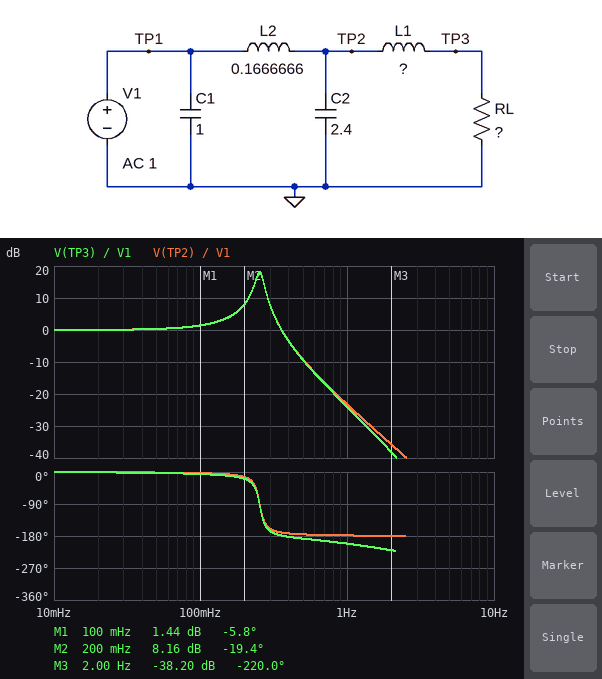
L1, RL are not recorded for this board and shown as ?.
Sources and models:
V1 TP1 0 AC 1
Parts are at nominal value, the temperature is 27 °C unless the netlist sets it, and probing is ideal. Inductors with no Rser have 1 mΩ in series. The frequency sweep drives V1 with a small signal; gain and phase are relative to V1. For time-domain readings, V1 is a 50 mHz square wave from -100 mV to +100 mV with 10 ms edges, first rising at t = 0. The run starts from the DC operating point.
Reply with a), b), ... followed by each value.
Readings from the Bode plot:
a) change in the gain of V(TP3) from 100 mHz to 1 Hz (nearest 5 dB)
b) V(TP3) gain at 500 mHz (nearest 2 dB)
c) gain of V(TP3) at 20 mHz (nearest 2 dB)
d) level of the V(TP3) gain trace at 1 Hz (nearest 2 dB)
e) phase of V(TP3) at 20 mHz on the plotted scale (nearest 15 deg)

a) -25 dB
b) -10 dB
c) 0 dB
d) -24 dB
e) 0 deg
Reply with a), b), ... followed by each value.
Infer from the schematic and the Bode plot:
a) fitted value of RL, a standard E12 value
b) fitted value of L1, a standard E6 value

a) 2.2 Ω
b) 150 mH
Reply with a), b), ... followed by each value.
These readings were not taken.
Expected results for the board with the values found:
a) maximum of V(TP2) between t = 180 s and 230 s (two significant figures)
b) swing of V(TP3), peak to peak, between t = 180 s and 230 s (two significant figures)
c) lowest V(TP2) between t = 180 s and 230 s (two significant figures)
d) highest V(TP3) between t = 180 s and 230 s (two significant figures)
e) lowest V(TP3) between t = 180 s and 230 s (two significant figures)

a) 360 mV
b) 720 mV
c) -360 mV
d) 360 mV
e) -360 mV
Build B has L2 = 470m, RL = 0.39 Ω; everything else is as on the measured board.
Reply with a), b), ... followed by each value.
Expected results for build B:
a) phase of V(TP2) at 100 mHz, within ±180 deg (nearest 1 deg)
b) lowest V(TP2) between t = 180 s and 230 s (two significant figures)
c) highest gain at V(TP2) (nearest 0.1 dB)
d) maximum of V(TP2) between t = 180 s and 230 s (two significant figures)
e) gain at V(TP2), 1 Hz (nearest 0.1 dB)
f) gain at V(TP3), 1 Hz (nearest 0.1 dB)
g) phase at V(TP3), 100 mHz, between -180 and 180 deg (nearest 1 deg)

a) -44 deg
b) -110 mV
c) 0 dB
d) 110 mV
e) -32.2 dB
f) -40.6 dB
g) -58 deg
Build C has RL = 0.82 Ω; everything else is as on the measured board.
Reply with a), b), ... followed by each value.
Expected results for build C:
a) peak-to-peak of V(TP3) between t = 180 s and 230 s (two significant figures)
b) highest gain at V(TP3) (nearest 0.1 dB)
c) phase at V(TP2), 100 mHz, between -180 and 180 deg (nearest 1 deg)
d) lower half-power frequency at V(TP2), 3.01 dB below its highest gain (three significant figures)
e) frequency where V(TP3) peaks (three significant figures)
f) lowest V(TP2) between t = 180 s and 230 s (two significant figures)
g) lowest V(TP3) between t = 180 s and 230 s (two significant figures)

a) 450 mV
b) 9.8 dB
c) -8 deg
d) 212 mHz
e) 257 mHz
f) -230 mV
g) -220 mV
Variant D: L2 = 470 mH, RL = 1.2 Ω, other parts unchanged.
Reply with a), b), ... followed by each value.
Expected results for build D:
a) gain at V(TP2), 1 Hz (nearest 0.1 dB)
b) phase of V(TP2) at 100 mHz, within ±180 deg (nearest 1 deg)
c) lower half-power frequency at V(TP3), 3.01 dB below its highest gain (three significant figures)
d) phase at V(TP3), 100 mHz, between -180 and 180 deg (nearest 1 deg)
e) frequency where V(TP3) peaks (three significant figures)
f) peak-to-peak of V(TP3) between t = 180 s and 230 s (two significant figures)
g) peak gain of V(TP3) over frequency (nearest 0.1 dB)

a) -32.5 dB
b) -23 deg
c) 115 mHz
d) -28 deg
e) 148 mHz
f) 460 mV
g) 8.6 dB
